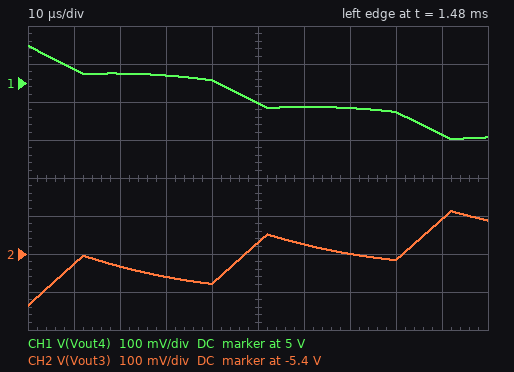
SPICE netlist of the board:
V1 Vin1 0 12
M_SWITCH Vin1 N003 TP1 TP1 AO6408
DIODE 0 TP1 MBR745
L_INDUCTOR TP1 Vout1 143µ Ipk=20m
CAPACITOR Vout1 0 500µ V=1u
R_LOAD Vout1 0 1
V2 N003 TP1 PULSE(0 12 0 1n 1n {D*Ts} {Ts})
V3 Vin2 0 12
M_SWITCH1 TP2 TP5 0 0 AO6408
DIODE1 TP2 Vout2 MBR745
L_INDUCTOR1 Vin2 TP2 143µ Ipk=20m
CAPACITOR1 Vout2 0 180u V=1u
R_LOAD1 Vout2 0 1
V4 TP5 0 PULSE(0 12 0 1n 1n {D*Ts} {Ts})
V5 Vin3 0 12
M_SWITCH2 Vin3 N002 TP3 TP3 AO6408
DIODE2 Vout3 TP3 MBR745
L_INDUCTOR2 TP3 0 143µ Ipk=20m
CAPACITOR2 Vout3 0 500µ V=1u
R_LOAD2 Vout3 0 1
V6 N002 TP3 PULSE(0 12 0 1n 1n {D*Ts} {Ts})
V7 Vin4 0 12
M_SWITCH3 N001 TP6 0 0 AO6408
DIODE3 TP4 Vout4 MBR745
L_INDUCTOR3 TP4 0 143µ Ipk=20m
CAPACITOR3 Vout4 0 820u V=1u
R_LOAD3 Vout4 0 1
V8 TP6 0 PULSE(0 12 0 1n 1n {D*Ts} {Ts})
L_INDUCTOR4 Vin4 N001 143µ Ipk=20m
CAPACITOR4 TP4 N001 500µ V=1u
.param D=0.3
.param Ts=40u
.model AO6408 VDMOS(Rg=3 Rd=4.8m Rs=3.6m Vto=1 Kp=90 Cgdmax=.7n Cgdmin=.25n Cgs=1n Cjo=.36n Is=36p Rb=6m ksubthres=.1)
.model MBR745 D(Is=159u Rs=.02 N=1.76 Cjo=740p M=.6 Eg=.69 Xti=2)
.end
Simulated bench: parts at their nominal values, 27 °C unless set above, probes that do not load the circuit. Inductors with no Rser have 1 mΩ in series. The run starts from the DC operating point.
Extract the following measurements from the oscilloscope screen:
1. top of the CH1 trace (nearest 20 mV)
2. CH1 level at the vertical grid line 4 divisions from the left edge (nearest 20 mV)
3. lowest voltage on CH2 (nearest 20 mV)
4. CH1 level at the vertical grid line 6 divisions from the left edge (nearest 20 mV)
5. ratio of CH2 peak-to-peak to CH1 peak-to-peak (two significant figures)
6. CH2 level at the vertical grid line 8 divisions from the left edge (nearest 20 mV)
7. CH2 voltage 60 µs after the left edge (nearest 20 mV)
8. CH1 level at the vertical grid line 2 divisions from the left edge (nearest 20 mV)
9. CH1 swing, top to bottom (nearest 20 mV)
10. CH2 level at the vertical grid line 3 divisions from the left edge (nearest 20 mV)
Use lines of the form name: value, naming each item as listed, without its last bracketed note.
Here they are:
top of the CH1 trace: 5.10 V
CH1 level at the vertical grid line 4 divisions from the left edge: 5.00 V
lowest voltage on CH2: -5.54 V
CH1 level at the vertical grid line 6 divisions from the left edge: 4.94 V
ratio of CH2 peak-to-peak to CH1 peak-to-peak: 1.0
CH2 level at the vertical grid line 8 divisions from the left edge: -5.42 V
CH2 voltage 60 µs after the left edge: -5.38 V
CH1 level at the vertical grid line 2 divisions from the left edge: 5.02 V
CH1 swing, top to bottom: 240 mV
CH2 level at the vertical grid line 3 divisions from the left edge: -5.46 V
